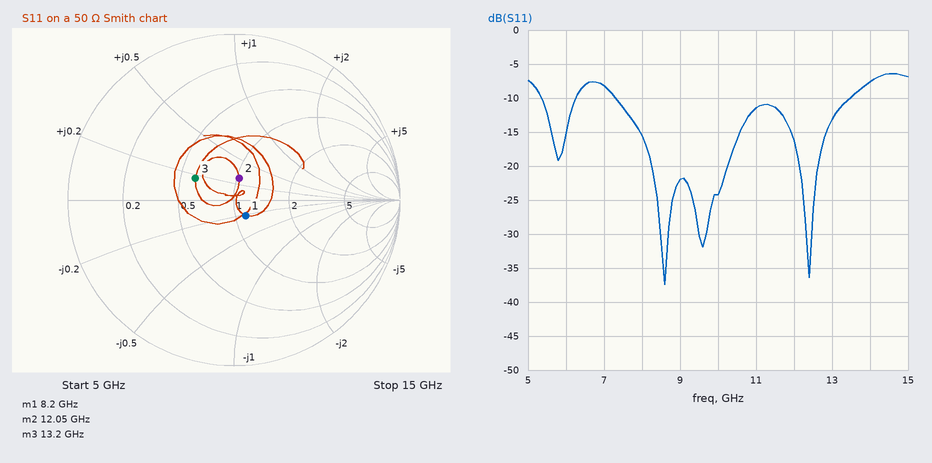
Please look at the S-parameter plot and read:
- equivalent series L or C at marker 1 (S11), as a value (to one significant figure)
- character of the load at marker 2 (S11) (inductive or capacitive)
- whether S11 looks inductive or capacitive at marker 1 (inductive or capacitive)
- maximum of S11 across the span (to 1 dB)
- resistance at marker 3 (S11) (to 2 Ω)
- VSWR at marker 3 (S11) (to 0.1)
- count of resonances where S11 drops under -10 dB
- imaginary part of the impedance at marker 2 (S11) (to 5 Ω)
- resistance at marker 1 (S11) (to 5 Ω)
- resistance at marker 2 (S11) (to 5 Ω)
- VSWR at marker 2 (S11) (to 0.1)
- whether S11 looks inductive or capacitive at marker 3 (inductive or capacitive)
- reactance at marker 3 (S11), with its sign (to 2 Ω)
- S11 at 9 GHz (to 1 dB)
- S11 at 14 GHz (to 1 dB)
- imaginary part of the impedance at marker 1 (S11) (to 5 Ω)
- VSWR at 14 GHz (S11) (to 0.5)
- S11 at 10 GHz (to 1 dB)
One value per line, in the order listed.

2 pF
inductive
capacitive
-6 dB
30 Ω
1.7
4
+15 Ω
55 Ω
50 Ω
1.3
inductive
+8 Ω
-22 dB
-8 dB
-10 Ω
2.5
-24 dB
